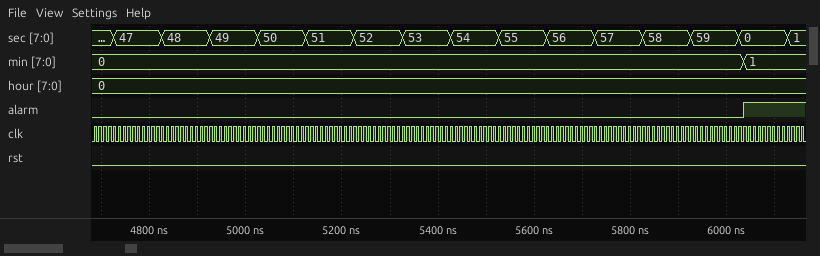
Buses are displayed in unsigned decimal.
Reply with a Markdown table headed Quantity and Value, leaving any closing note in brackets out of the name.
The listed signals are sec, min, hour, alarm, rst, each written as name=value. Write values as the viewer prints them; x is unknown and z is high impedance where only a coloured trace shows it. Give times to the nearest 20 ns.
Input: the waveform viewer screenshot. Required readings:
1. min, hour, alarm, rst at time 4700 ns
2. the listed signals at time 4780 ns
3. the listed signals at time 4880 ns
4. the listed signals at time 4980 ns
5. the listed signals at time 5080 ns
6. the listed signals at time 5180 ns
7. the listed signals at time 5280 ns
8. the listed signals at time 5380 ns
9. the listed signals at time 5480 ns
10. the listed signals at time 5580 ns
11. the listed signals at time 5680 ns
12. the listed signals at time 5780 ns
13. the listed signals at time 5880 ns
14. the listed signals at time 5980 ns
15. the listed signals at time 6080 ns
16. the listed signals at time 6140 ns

| Quantity | Value |
|---|---|
| min, hour, alarm, rst at time 4700 ns | min=0, hour=0, alarm=0, rst=0 |
| the listed signals at time 4780 ns | sec=47, min=0, hour=0, alarm=0, rst=0 |
| the listed signals at time 4880 ns | sec=48, min=0, hour=0, alarm=0, rst=0 |
| the listed signals at time 4980 ns | sec=49, min=0, hour=0, alarm=0, rst=0 |
| the listed signals at time 5080 ns | sec=50, min=0, hour=0, alarm=0, rst=0 |
| the listed signals at time 5180 ns | sec=51, min=0, hour=0, alarm=0, rst=0 |
| the listed signals at time 5280 ns | sec=52, min=0, hour=0, alarm=0, rst=0 |
| the listed signals at time 5380 ns | sec=53, min=0, hour=0, alarm=0, rst=0 |
| the listed signals at time 5480 ns | sec=54, min=0, hour=0, alarm=0, rst=0 |
| the listed signals at time 5580 ns | sec=55, min=0, hour=0, alarm=0, rst=0 |
| the listed signals at time 5680 ns | sec=56, min=0, hour=0, alarm=0, rst=0 |
| the listed signals at time 5780 ns | sec=57, min=0, hour=0, alarm=0, rst=0 |
| the listed signals at time 5880 ns | sec=58, min=0, hour=0, alarm=0, rst=0 |
| the listed signals at time 5980 ns | sec=59, min=0, hour=0, alarm=0, rst=0 |
| the listed signals at time 6080 ns | sec=0, min=1, hour=0, alarm=1, rst=0 |
| the listed signals at time 6140 ns | sec=1, min=1, hour=0, alarm=1, rst=0 |
